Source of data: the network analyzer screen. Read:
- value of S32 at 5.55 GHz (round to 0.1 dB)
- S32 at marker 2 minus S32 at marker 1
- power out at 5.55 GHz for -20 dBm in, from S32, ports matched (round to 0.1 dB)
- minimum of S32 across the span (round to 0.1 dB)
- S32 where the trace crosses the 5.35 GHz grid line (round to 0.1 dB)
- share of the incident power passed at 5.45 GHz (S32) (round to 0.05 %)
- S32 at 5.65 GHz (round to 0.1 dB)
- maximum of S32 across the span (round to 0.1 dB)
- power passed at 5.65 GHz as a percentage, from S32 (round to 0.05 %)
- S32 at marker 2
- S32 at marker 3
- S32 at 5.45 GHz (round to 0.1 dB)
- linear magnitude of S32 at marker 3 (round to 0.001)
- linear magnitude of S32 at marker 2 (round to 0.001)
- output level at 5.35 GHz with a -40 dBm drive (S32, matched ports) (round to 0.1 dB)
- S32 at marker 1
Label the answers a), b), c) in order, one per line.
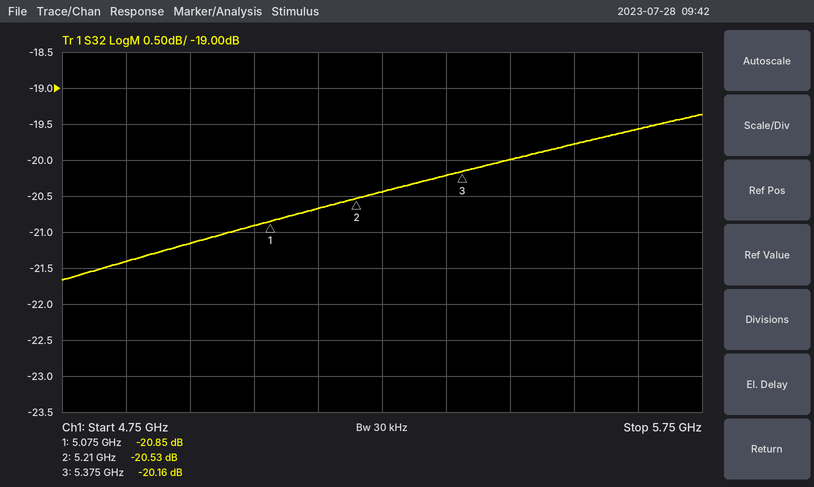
a) -19.8 dB
b) 0.32 dB
c) -39.8 dBm
d) -21.7 dB
e) -20.2 dB
f) 1.00 %
g) -19.6 dB
h) -19.4 dB
i) 1.10 %
j) -20.53 dB
k) -20.16 dB
l) -20.0 dB
m) 0.098
n) 0.094
o) -60.2 dBm
p) -20.85 dB
